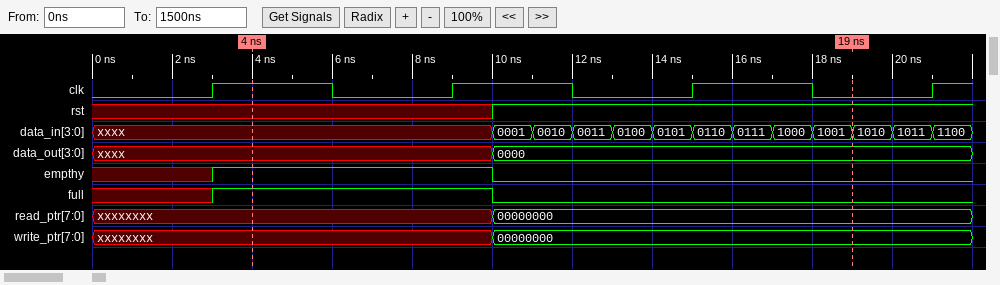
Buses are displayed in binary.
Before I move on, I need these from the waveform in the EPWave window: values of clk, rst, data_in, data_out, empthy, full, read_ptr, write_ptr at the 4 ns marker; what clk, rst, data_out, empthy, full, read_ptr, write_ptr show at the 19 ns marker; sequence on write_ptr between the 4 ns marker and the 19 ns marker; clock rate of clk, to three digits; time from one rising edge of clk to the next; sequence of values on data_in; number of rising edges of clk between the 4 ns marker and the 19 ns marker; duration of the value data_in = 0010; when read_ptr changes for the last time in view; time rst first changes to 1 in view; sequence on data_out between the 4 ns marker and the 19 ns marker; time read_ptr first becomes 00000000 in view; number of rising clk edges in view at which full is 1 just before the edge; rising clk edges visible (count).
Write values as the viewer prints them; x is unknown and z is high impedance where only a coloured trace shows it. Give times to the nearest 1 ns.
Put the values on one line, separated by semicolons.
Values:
clk=1, rst=x, data_in=xxxx, data_out=xxxx, empthy=1, full=1, read_ptr=xxxxxxxx, write_ptr=xxxxxxxx; clk=0, rst=1, data_out=0000, empthy=0, full=0, read_ptr=00000000, write_ptr=00000000; xxxxxxxx, 00000000; 167 MHz; 6 ns; xxxx, 0001, 0010, 0011, 0100, 0101, 0110, 0111, 1000, 1001, 1010, 1011, 1100; 2; 1 ns; 10 ns; 10 ns; xxxx, 0000; 10 ns; 1; 4
